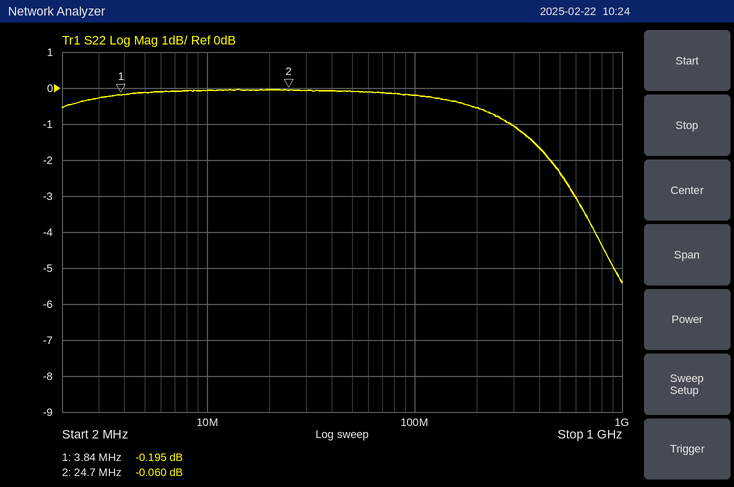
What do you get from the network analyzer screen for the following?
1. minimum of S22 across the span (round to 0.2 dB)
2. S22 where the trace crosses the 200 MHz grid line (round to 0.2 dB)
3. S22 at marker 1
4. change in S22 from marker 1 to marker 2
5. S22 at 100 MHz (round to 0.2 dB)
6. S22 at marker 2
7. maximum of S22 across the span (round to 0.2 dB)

-5.4 dB
-0.6 dB
-0.195 dB
0.135 dB
-0.2 dB
-0.060 dB
0.0 dB
